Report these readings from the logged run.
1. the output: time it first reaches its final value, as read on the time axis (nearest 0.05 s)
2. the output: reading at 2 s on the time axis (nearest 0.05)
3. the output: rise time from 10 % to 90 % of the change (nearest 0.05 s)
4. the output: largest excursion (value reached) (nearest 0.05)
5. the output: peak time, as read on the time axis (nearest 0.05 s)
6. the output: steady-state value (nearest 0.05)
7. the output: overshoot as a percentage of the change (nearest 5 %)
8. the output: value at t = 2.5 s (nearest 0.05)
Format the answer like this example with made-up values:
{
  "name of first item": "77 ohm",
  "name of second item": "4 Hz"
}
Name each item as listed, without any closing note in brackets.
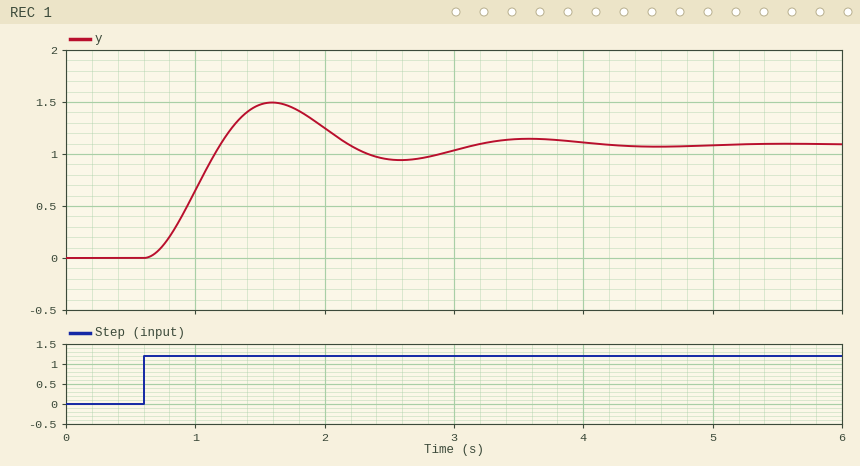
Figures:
{
  "the output: time it first reaches its final value, as read on the time axis": "1.20 s",
  "the output: reading at 2 s on the time axis": "1.25",
  "the output: rise time from 10 % to 90 % of the change": "0.40 s",
  "the output: largest excursion (value reached)": "1.50",
  "the output: peak time, as read on the time axis": "1.60 s",
  "the output: steady-state value": "1.10",
  "the output: overshoot as a percentage of the change": "35 %",
  "the output: value at t = 2.5 s": "0.95"
}
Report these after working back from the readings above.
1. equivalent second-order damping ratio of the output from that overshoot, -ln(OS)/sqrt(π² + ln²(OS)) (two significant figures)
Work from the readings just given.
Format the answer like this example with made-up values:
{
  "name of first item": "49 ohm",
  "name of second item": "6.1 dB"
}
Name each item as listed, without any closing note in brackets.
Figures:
{
  "equivalent second-order damping ratio of the output from that overshoot, -ln(OS)/sqrt(π² + ln²(OS))": "0.32"
}
